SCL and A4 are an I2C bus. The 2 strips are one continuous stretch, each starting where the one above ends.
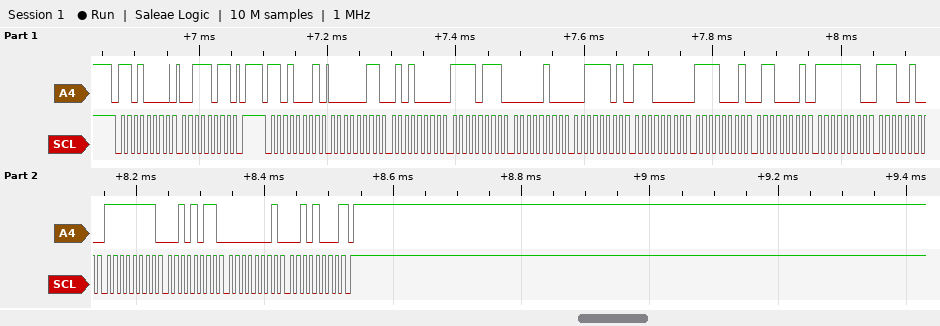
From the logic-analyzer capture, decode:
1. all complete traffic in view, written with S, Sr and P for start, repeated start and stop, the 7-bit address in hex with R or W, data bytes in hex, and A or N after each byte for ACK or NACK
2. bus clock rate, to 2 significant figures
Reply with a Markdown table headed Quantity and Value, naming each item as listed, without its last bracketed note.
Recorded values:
| Quantity | Value |
|---|---|
| all complete traffic in view, written with S, Sr and P for start, repeated start and stop, the 7-bit address in hex with R or W, data bytes in hex, and A or N after each byte for ACK or NACK | S 68W A 3B A P S 68R A 03 A 50 A F7 A 04 A 3D A E0 A F1 A 61 A FE A E4 A FF A 2B A 01 A 28 N P |
| bus clock rate, to 2 significant figures | 100 kHz |
